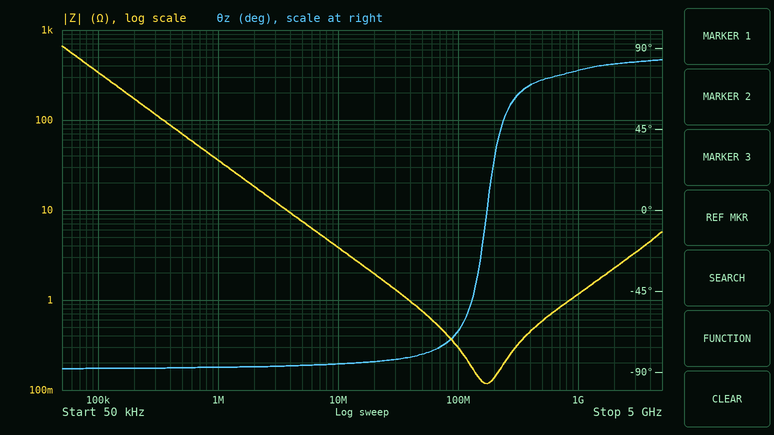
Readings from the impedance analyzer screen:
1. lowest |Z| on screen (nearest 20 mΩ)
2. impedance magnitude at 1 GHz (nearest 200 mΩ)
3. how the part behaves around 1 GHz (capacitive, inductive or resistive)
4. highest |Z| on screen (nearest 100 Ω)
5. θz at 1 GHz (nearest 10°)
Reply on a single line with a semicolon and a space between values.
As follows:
120 mΩ; 1.2 Ω; inductive; 700 Ω; 80°
